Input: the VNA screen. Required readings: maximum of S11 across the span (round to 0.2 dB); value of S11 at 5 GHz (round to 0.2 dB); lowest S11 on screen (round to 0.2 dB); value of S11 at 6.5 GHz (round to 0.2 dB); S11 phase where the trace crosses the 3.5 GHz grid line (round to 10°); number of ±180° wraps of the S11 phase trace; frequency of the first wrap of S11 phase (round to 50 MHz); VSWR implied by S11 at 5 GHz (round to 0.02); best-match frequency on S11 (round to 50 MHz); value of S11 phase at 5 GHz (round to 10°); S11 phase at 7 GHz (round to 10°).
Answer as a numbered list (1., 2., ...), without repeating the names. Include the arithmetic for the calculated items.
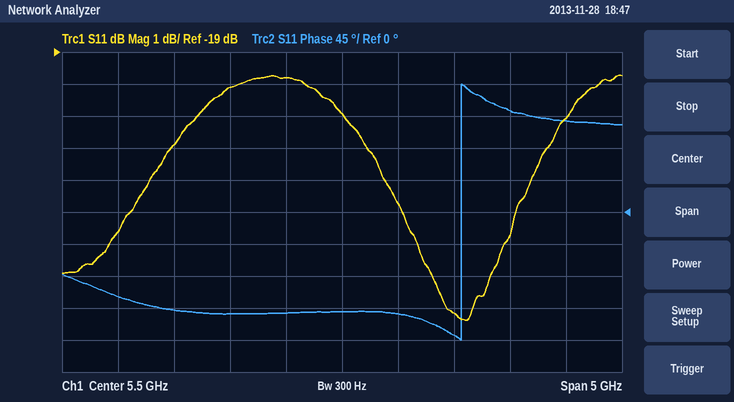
1. -19.8 dB
2. -19.8 dB
3. -27.4 dB
4. -27.2 dB
5. -120°
6. 1
7. 6.55 GHz
8. |Γ| = 10^(-19.8/20) = 0.1023; VSWR = (1 + 0.1023)/(1 − 0.1023) ≈ 1.23, so 1.22 to the nearest 0.02
9. 6.60 GHz
10. -140°
11. 140°
